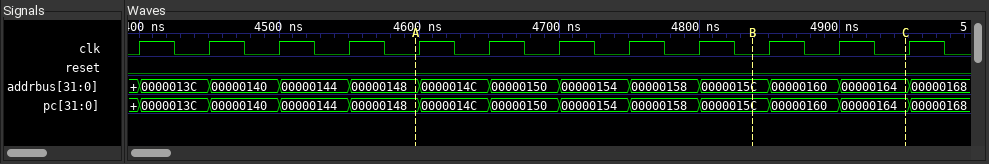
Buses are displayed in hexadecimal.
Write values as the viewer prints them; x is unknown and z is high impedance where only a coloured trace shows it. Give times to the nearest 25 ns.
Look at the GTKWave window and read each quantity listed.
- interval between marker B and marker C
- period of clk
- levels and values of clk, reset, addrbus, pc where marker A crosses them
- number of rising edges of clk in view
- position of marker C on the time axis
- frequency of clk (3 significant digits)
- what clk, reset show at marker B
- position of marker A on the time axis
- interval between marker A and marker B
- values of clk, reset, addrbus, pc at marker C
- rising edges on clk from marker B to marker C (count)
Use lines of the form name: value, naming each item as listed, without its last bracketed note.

interval between marker B and marker C: 100 ns
period of clk: 50 ns
levels and values of clk, reset, addrbus, pc where marker A crosses them: clk=0, reset=0, addrbus=00000148, pc=00000148
number of rising edges of clk in view: 12
position of marker C on the time axis: 4950 ns
frequency of clk: 20.0 MHz
what clk, reset show at marker B: clk=0, reset=0
position of marker A on the time axis: 4600 ns
interval between marker A and marker B: 250 ns
values of clk, reset, addrbus, pc at marker C: clk=0, reset=0, addrbus=00000164, pc=00000164
rising edges on clk from marker B to marker C: 2
